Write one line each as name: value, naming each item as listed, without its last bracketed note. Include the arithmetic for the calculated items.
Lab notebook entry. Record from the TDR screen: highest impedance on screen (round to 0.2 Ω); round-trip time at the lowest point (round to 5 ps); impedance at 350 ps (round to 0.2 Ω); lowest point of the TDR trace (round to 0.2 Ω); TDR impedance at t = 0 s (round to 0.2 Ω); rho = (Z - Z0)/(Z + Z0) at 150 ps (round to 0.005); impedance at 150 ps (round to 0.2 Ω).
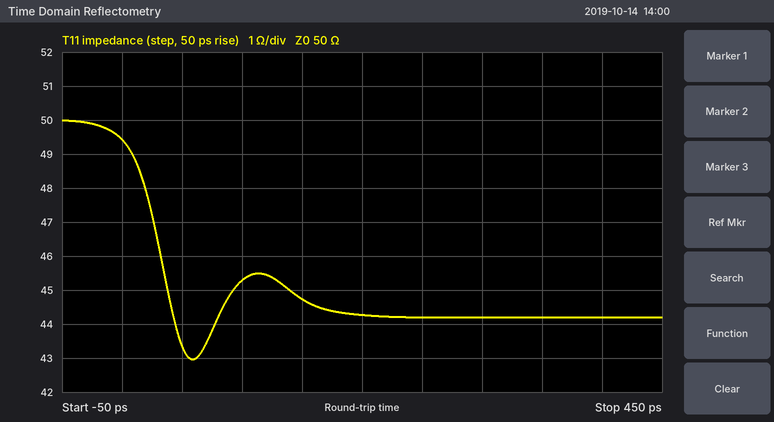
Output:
highest impedance on screen: 50.0 Ω
round-trip time at the lowest point: 60 ps
impedance at 350 ps: 44.2 Ω
lowest point of the TDR trace: 43.0 Ω
TDR impedance at t = 0 s: 49.4 Ω
rho = (Z - Z0)/(Z + Z0) at 150 ps: (44.8 − 50)/(44.8 + 50) ≈ -0.055
impedance at 150 ps: 44.8 Ω
